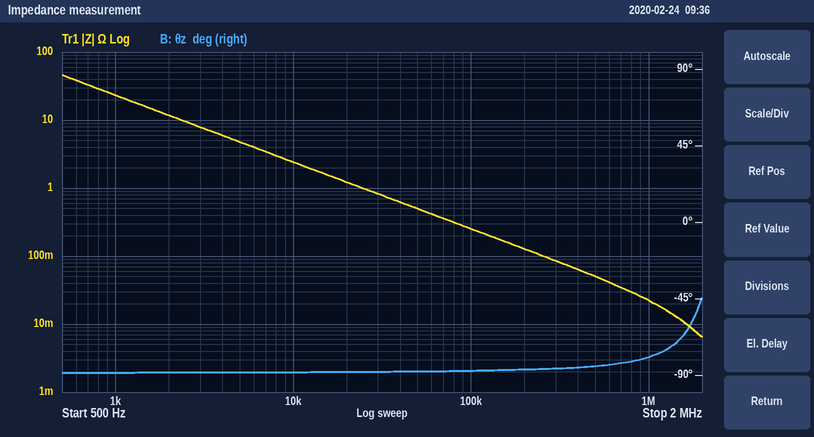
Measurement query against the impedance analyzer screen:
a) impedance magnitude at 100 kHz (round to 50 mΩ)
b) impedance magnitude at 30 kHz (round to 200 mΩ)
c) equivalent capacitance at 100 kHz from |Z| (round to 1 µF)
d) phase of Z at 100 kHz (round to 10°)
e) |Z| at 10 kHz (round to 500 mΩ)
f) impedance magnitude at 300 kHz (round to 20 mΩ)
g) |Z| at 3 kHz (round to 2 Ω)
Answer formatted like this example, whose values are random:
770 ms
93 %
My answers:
250 mΩ
800 mΩ
6 µF
-90°
2.5 Ω
80 mΩ
8 Ω
